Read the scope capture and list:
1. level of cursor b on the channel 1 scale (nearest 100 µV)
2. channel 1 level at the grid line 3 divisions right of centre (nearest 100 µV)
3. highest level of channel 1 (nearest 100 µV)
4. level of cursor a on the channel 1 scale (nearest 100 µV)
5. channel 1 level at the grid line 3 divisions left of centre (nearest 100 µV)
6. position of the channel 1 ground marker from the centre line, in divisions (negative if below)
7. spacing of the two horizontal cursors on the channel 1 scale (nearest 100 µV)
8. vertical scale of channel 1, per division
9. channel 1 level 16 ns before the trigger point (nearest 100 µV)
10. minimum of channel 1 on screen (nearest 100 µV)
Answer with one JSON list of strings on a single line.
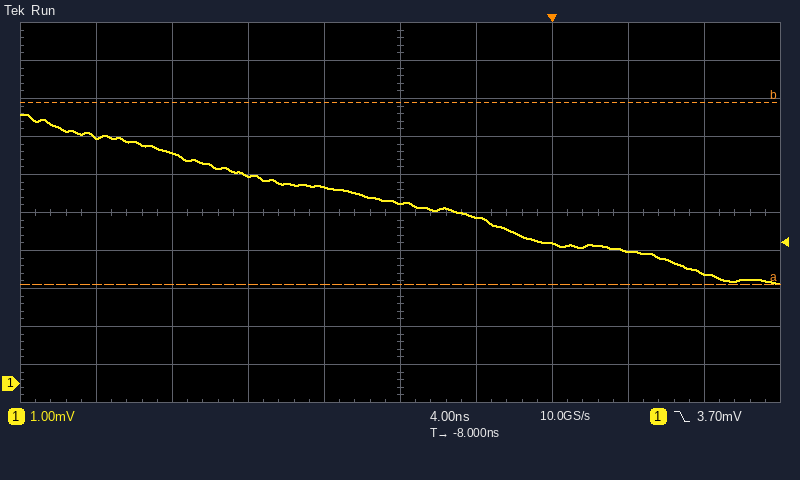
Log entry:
["7.4 mV", "3.5 mV", "7.1 mV", "2.6 mV", "6.1 mV", "-4.5 div", "4.8 mV", "1 mV", "5.5 mV", "2.6 mV"]
